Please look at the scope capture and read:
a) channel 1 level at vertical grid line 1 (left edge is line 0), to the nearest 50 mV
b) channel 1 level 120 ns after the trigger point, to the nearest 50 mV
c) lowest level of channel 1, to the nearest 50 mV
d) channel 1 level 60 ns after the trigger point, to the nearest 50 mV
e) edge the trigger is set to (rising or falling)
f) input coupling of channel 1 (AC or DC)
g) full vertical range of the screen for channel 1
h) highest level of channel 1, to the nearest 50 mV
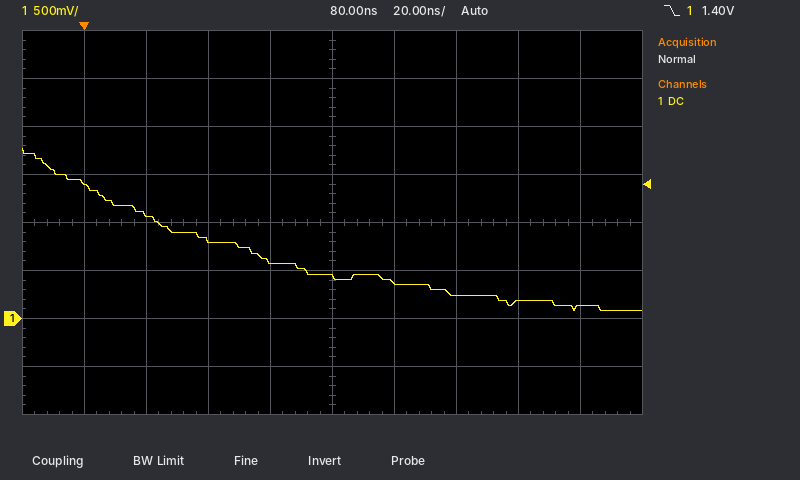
1.40 V
250 mV
100 mV
600 mV
falling
DC
4 V
1.75 V
